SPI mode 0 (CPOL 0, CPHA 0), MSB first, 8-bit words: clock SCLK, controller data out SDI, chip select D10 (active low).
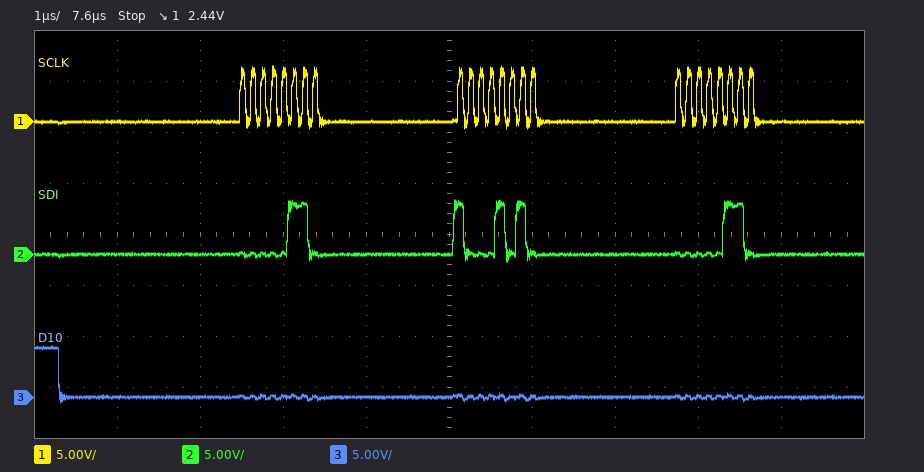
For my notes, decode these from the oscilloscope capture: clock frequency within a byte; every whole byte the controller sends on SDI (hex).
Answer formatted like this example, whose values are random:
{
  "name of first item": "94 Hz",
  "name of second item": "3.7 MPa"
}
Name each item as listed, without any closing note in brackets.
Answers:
{
  "clock frequency within a byte": "8 MHz",
  "every whole byte the controller sends on SDI": "06 8A 06"
}
